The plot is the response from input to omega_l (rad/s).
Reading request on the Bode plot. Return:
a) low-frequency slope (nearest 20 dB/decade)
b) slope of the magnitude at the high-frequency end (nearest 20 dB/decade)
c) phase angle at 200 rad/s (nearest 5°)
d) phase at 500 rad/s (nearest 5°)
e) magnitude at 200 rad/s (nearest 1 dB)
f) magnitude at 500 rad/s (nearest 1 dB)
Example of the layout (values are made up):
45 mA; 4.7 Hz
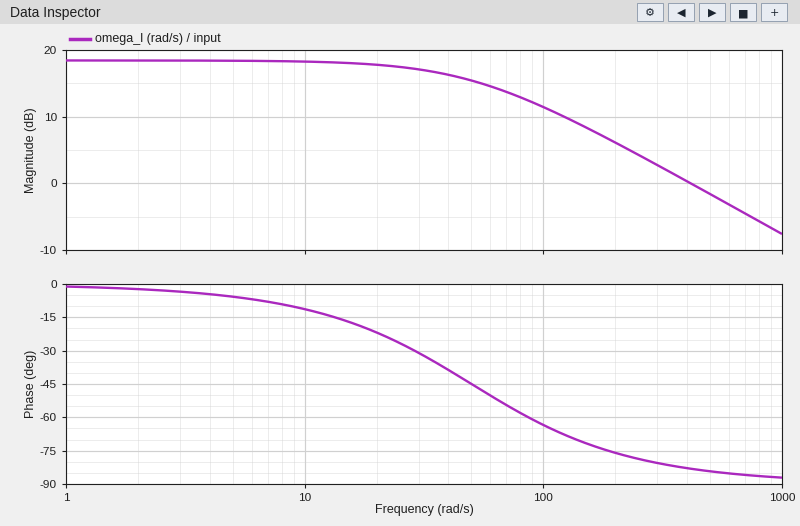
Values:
0 dB/decade; -20 dB/decade; -75°; -85°; 6 dB; -2 dB
